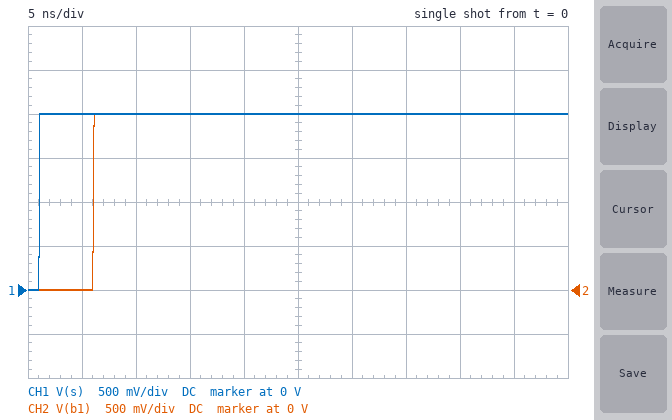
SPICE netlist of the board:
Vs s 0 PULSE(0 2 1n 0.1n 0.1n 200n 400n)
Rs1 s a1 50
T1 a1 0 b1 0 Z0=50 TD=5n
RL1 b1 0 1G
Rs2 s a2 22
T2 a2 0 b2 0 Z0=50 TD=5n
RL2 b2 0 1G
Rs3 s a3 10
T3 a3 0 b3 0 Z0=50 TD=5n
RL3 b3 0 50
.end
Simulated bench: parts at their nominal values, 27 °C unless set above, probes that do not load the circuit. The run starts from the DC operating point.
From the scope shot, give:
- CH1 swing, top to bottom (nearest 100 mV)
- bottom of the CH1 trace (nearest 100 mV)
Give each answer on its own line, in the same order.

2.0 V
0 V
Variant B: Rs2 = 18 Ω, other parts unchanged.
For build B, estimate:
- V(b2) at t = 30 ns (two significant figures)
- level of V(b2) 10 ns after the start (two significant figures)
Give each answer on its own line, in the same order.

2.2 V
2.9 V
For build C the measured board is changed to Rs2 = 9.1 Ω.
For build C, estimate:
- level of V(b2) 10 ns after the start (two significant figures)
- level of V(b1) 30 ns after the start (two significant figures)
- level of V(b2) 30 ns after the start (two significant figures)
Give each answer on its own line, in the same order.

3.4 V
2.0 V
2.7 V
